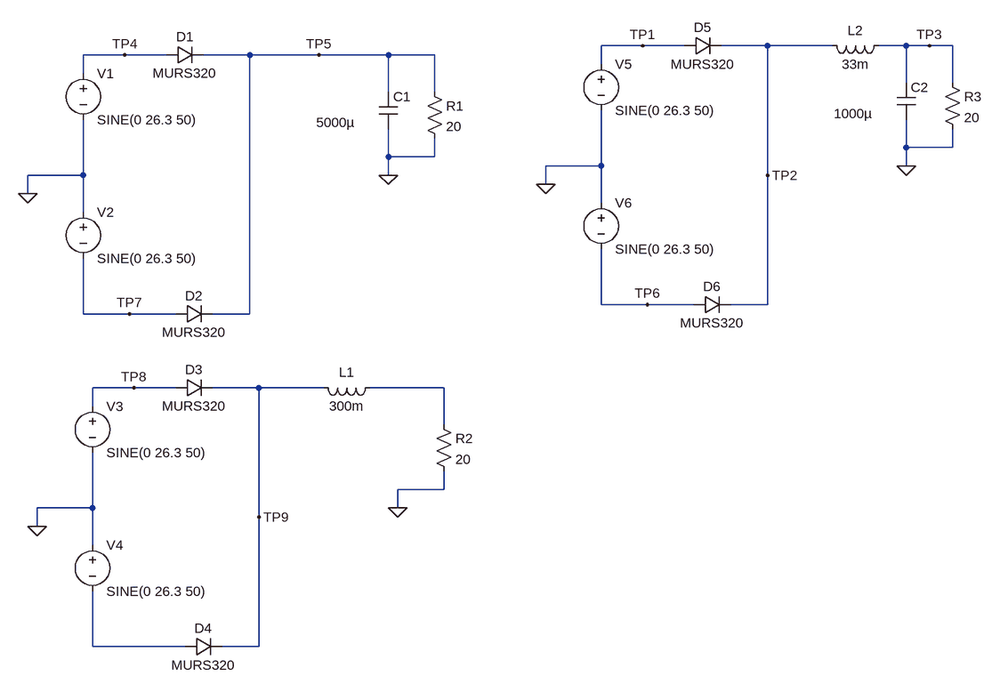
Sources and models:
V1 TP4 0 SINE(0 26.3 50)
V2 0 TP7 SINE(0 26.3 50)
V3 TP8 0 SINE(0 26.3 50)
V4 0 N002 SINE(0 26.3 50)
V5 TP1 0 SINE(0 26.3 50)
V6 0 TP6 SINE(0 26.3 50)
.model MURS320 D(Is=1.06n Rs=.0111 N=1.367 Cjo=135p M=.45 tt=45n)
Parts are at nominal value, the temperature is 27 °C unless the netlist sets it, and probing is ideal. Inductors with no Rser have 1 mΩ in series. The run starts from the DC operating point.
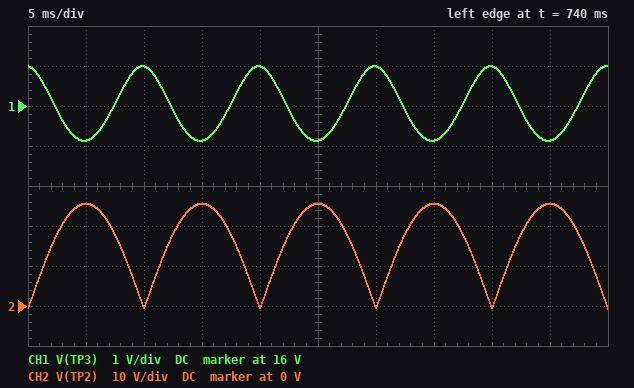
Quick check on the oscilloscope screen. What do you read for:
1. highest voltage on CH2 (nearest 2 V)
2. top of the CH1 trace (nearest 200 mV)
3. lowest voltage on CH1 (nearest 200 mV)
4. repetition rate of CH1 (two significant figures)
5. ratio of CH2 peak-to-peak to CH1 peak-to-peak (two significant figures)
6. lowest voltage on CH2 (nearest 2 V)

26 V
17.0 V
15.2 V
100 Hz
14
0 V
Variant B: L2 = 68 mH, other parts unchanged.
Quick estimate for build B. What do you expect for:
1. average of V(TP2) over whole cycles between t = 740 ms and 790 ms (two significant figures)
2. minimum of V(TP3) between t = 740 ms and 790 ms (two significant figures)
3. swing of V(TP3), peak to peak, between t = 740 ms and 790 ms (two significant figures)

16 V
16 V
870 mV
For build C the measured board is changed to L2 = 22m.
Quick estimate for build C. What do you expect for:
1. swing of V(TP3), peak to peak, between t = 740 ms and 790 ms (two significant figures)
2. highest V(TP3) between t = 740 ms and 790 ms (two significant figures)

2.8 V
18 V
